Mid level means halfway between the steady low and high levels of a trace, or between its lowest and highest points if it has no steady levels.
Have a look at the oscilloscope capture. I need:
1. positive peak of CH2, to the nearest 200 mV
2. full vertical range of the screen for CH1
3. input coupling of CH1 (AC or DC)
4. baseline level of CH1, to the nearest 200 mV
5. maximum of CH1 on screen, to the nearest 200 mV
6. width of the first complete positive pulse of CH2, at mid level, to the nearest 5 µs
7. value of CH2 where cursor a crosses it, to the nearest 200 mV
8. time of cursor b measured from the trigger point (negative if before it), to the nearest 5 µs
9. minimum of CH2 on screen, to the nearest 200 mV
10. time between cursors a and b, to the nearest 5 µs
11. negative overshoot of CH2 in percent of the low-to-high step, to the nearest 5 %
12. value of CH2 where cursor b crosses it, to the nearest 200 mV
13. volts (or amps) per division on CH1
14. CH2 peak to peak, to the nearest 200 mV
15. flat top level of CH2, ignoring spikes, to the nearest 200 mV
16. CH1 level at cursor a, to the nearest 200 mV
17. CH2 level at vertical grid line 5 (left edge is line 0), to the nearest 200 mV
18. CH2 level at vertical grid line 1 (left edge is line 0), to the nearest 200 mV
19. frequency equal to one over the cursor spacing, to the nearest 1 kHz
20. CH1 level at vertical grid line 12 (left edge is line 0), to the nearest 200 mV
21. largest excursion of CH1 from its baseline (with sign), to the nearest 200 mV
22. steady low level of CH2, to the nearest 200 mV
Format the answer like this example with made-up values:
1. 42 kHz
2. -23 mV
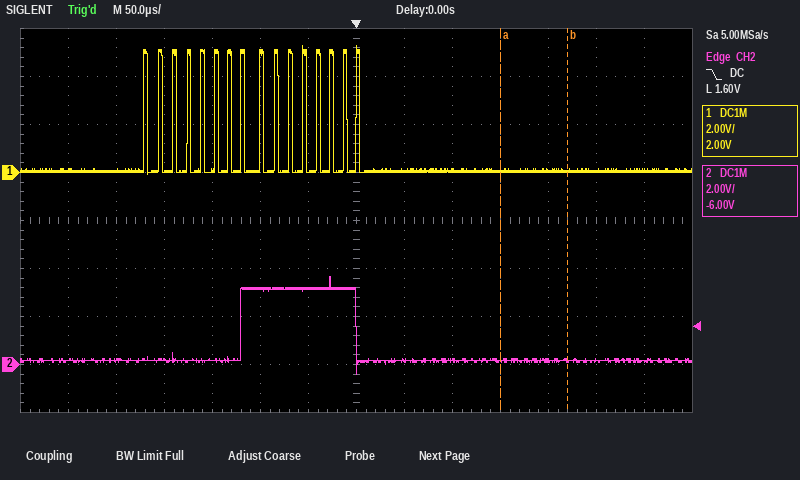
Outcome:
1. 3.6 V
2. 16 V
3. DC
4. 0.0 V
5. 5.2 V
6. 120 µs
7. 200 mV
8. +220 µs
9. -400 mV
10. 70 µs
11. 20 %
12. 200 mV
13. 2 V
14. 4.0 V
15. 3.2 V
16. 0.0 V
17. 3.2 V
18. 200 mV
19. 14 kHz
20. 0.0 V
21. +5.2 V
22. 200 mV
